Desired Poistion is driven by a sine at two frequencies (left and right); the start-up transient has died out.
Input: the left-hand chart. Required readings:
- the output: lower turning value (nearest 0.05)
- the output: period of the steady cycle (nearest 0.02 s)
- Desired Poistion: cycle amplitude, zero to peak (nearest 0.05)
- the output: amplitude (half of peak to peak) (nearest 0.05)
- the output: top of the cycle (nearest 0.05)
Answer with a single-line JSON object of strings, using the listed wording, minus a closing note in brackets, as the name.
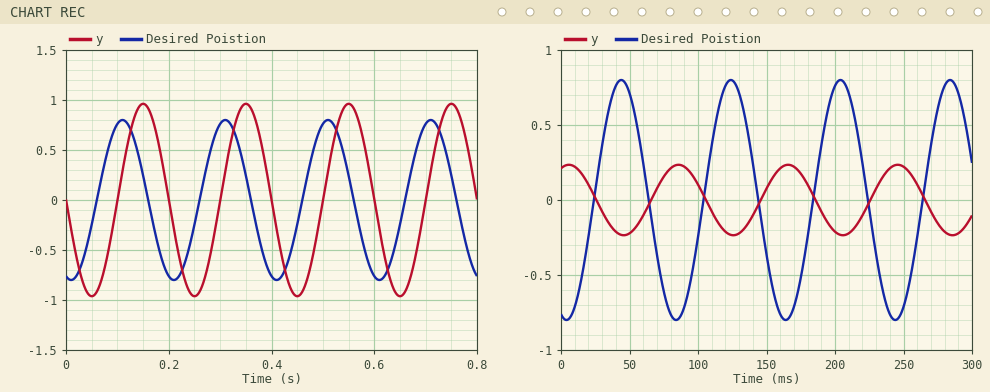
{"the output: lower turning value": "-0.95", "the output: period of the steady cycle": "0.20 s", "Desired Poistion: cycle amplitude, zero to peak": "0.80", "the output: amplitude (half of peak to peak)": "0.95", "the output: top of the cycle": "0.95"}
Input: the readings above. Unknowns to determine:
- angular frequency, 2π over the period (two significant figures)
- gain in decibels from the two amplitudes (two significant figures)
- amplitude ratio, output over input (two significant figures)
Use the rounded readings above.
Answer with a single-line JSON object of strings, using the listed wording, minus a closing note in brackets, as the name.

{"angular frequency, 2π over the period": "31 rad/s", "gain in decibels from the two amplitudes": "1.5 dB", "amplitude ratio, output over input": "1.2"}
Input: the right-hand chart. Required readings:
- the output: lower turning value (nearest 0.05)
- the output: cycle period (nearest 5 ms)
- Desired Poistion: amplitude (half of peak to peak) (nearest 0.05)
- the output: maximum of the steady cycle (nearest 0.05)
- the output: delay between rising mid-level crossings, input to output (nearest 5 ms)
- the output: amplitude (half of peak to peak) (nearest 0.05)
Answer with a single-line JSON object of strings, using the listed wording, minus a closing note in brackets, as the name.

{"the output: lower turning value": "-0.25", "the output: cycle period": "80 ms", "Desired Poistion: amplitude (half of peak to peak)": "0.80", "the output: maximum of the steady cycle": "0.25", "the output: delay between rising mid-level crossings, input to output": "40 ms", "the output: amplitude (half of peak to peak)": "0.25"}
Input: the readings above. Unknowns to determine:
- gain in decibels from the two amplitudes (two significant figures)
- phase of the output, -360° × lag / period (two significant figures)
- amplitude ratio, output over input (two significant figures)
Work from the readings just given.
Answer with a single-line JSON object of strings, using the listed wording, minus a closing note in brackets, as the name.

{"gain in decibels from the two amplitudes": "-10 dB", "phase of the output, -360° × lag / period": "-180°", "amplitude ratio, output over input": "0.31"}
